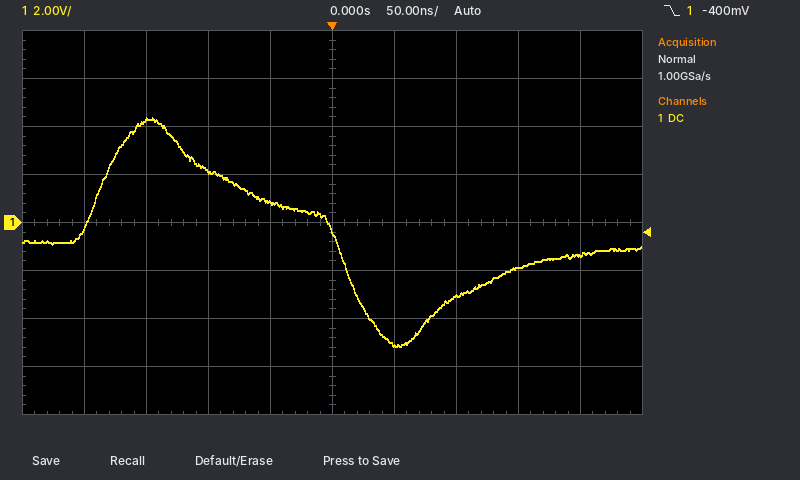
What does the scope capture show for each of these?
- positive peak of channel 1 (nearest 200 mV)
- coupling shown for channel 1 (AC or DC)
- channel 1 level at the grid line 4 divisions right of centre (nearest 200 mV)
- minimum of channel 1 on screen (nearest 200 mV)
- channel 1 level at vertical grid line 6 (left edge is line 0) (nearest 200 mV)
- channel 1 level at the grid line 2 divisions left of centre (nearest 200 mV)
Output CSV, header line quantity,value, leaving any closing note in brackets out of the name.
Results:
quantity,value
positive peak of channel 1,4.4 V
coupling shown for channel 1,DC
channel 1 level at the grid line 4 divisions right of centre,-1.4 V
minimum of channel 1 on screen,-5.2 V
channel 1 level at vertical grid line 6 (left edge is line 0),-5.0 V
channel 1 level at the grid line 2 divisions left of centre,2.2 V
